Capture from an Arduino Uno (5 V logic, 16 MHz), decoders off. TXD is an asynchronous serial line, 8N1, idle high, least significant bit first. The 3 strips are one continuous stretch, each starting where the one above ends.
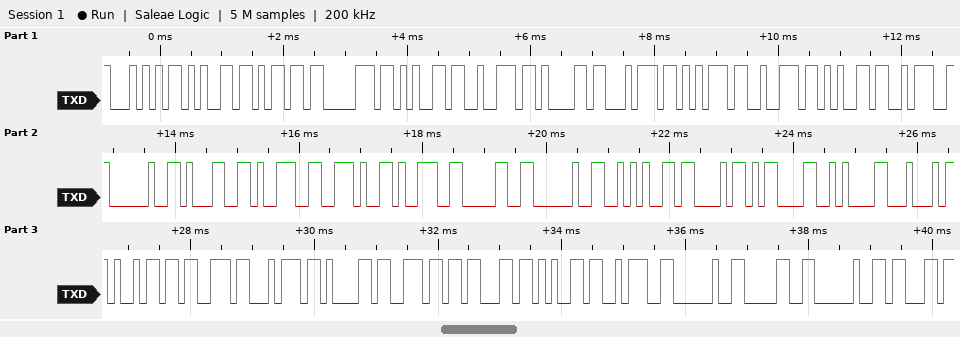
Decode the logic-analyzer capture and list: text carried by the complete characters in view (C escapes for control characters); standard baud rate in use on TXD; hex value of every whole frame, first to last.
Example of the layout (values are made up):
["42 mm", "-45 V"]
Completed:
["\"Temperature: 19.90 *C\\r\\nDistance: 0 c\"", "9600 baud", "54 65 6D 70 65 72 61 74 75 72 65 3A 20 31 39 2E 39 30 20 2A 43 0D 0A 44 69 73 74 61 6E 63 65 3A 20 30 20 63"]
